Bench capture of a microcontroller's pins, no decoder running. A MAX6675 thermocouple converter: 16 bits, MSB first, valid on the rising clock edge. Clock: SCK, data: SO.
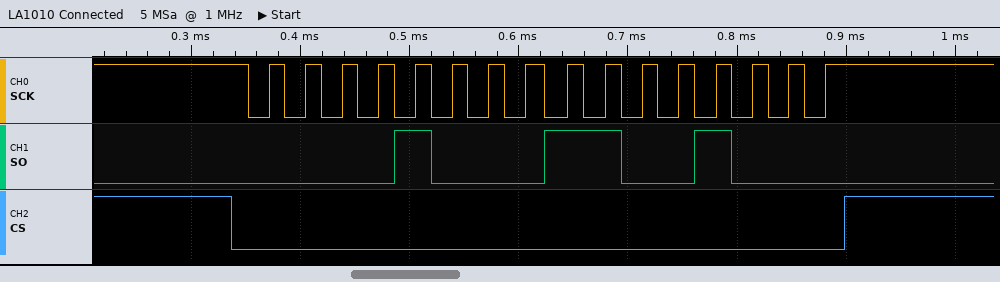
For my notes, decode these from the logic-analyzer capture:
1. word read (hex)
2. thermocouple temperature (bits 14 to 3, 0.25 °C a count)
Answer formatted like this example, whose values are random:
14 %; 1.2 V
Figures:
0x08C8; 70.25 °C
